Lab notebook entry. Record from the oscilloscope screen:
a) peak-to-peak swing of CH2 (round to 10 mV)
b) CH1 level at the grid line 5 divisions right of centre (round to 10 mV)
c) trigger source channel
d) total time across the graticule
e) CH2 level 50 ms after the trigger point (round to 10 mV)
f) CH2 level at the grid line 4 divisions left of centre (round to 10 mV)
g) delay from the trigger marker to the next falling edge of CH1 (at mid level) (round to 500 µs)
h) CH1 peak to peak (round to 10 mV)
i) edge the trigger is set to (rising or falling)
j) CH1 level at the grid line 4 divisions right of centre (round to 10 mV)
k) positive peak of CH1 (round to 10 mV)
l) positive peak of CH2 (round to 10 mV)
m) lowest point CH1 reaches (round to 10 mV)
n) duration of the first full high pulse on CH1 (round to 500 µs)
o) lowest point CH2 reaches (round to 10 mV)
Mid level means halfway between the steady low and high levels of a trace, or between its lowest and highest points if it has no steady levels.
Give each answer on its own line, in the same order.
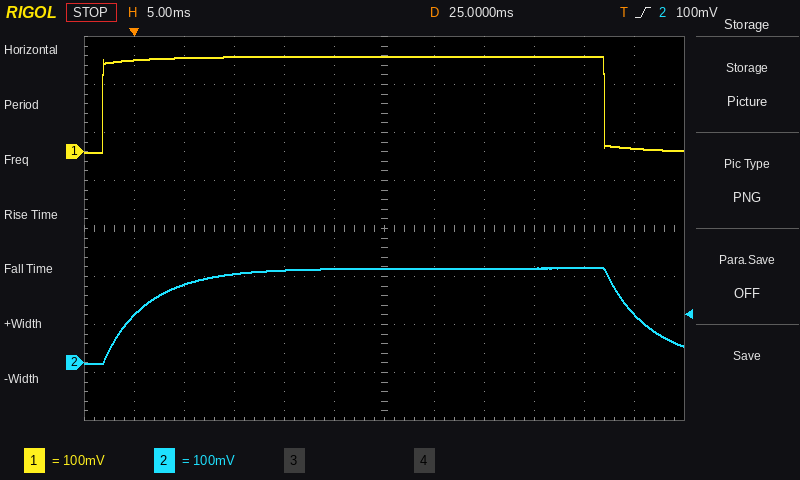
200 mV
10 mV
CH2
60 ms
100 mV
160 mV
47.0 ms
200 mV
rising
200 mV
200 mV
200 mV
0 mV
50.0 ms
0 mV
